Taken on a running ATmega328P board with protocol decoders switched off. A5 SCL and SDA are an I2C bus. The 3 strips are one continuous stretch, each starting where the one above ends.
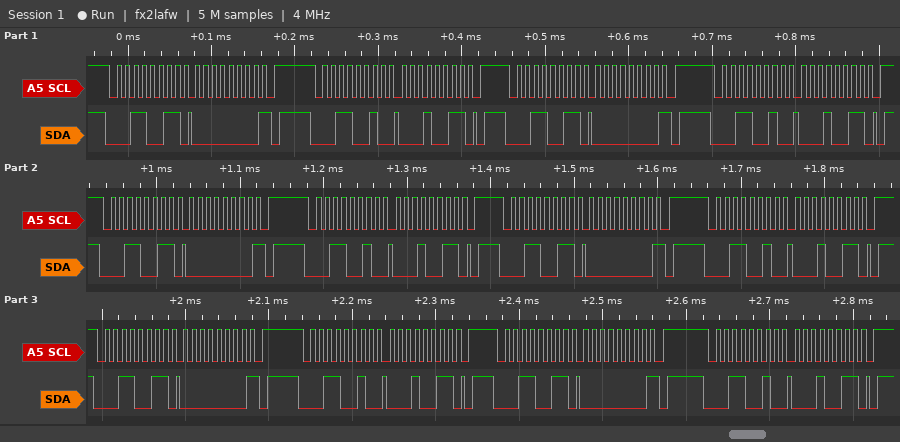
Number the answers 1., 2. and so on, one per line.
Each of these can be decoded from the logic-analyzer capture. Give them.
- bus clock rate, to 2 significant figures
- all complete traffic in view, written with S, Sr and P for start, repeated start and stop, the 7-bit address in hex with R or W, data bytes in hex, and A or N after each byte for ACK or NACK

1. 100 kHz
2. S 19R A 00 N P S 19W A 13 A P S 19R A 00 N P S 19W A 13 A P S 19R A 00 N P S 19W A 13 A P S 19R A 00 N P S 19W A 13 A P S 19R A 00 N P S 19W A 13 A P S 19R A 00 N P S 19W A 13 A P
